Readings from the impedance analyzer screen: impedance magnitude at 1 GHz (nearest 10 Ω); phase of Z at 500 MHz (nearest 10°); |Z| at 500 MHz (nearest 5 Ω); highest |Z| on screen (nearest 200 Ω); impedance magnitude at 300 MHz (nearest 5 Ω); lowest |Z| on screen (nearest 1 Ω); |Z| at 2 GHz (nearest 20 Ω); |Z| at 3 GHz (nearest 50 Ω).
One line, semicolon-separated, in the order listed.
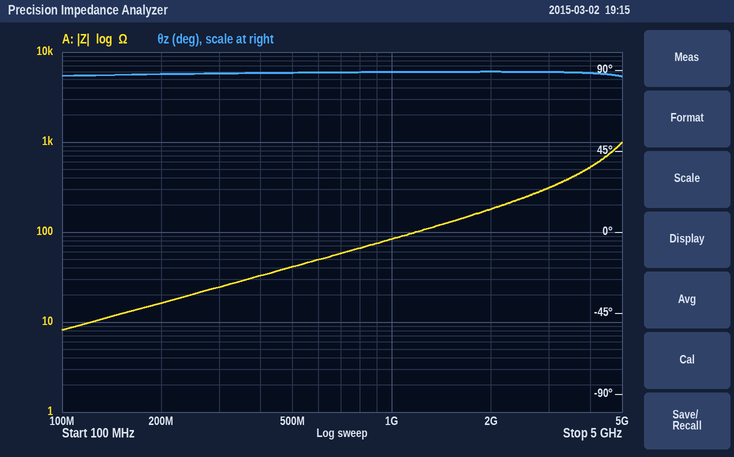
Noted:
80 Ω; 90°; 40 Ω; 1.0 kΩ; 25 Ω; 8 Ω; 180 Ω; 300 Ω
